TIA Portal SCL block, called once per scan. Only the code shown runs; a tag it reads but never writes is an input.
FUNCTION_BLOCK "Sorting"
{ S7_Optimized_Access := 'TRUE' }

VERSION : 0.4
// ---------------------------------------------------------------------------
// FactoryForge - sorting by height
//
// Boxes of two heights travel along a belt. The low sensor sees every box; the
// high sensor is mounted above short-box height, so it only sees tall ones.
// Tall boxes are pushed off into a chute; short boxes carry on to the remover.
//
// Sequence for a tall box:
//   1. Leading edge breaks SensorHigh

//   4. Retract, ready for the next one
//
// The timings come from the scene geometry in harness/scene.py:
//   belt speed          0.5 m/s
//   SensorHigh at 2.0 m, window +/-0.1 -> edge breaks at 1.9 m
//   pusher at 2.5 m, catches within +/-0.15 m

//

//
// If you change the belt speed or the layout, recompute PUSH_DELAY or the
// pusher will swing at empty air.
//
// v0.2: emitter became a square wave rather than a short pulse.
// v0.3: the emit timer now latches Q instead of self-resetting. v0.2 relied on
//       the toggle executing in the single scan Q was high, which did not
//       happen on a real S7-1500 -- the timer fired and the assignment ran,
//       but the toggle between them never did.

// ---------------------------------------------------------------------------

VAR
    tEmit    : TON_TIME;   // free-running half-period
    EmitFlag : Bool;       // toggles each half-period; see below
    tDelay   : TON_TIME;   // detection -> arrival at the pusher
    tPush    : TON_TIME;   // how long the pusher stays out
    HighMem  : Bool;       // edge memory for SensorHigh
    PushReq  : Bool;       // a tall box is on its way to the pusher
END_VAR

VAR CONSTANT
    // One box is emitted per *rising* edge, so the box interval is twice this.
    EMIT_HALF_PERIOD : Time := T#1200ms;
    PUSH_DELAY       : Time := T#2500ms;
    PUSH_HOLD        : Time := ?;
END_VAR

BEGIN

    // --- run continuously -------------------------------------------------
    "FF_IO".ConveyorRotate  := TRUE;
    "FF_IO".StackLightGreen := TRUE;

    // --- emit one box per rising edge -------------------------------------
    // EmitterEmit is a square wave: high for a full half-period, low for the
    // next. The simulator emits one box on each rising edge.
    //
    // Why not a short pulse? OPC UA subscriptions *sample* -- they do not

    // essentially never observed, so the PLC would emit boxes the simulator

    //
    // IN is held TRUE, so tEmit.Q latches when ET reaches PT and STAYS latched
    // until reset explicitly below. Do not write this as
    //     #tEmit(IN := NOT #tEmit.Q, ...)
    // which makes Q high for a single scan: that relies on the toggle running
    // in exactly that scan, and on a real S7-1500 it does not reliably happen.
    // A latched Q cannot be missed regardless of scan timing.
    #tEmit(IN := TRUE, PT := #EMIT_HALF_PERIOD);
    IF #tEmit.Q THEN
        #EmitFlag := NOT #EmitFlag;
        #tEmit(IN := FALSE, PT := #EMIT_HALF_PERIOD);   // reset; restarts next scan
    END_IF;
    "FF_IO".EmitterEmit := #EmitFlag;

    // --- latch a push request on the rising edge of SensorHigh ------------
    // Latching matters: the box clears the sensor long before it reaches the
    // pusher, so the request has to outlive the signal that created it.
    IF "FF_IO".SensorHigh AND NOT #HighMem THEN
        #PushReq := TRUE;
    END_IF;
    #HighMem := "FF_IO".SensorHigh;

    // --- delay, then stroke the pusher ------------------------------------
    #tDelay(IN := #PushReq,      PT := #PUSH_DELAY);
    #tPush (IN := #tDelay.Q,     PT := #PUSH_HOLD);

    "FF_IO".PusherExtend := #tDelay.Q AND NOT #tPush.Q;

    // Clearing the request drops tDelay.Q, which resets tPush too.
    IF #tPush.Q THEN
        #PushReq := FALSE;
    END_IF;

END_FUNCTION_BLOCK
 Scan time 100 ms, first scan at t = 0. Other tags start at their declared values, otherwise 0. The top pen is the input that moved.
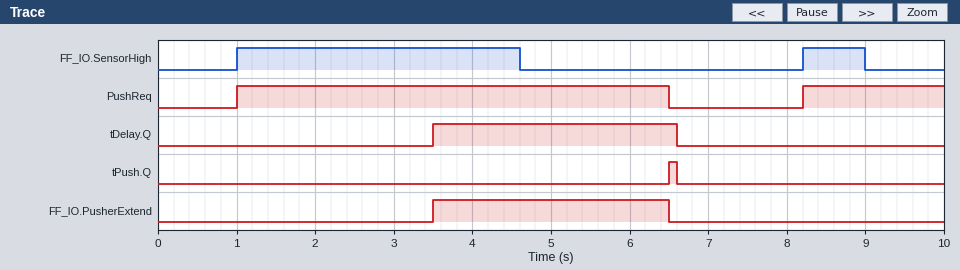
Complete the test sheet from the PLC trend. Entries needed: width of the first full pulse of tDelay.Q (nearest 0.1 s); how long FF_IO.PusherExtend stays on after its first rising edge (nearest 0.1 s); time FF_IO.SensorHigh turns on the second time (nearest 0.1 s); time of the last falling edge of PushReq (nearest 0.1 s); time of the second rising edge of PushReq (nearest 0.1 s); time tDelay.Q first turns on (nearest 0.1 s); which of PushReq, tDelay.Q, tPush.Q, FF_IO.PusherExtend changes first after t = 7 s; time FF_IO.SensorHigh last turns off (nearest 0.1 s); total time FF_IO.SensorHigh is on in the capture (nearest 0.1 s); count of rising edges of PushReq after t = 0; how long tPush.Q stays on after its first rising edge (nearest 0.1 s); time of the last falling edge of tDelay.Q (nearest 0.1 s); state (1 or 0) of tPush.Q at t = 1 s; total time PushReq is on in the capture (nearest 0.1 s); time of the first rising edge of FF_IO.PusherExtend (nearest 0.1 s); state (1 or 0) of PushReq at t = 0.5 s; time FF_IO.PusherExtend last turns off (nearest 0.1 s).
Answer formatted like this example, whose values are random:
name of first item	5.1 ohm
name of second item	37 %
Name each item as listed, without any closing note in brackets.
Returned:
width of the first full pulse of tDelay.Q	3.1 s
how long FF_IO.PusherExtend stays on after its first rising edge	3.0 s
time FF_IO.SensorHigh turns on the second time	8.2 s
time of the last falling edge of PushReq	6.5 s
time of the second rising edge of PushReq	8.2 s
time tDelay.Q first turns on	3.5 s
which of PushReq, tDelay.Q, tPush.Q, FF_IO.PusherExtend changes first after t = 7 s	PushReq
time FF_IO.SensorHigh last turns off	9.0 s
total time FF_IO.SensorHigh is on in the capture	4.4 s
count of rising edges of PushReq after t = 0	2
how long tPush.Q stays on after its first rising edge	0.1 s
time of the last falling edge of tDelay.Q	6.6 s
state (1 or 0) of tPush.Q at t = 1 s	0
total time PushReq is on in the capture	7.3 s
time of the first rising edge of FF_IO.PusherExtend	3.5 s
state (1 or 0) of PushReq at t = 0.5 s	0
time FF_IO.PusherExtend last turns off	6.5 s
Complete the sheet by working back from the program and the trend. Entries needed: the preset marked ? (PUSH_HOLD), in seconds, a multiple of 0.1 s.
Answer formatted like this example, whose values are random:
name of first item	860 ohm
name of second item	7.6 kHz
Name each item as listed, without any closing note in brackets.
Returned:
the preset marked ? (PUSH_HOLD), in seconds, a multiple of 0.1 s	3.0 s
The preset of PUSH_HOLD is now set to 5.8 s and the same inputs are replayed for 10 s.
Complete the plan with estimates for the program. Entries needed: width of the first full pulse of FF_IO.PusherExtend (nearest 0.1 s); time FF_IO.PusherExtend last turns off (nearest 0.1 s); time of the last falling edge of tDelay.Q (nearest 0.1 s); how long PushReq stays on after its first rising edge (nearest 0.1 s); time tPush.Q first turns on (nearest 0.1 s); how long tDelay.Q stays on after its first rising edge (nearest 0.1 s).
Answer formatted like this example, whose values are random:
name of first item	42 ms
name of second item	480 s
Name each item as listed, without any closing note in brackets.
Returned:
width of the first full pulse of FF_IO.PusherExtend	5.8 s
time FF_IO.PusherExtend last turns off	9.3 s
time of the last falling edge of tDelay.Q	9.4 s
how long PushReq stays on after its first rising edge	8.3 s
time tPush.Q first turns on	9.3 s
how long tDelay.Q stays on after its first rising edge	5.9 s
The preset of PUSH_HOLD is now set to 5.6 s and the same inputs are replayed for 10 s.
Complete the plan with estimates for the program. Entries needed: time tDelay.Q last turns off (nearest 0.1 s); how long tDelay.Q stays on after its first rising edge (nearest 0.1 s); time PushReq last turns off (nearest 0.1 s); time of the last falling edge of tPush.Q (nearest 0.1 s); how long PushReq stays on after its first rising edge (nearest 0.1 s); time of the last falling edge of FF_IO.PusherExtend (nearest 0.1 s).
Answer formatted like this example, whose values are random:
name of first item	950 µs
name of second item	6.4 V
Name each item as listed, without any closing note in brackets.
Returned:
time tDelay.Q last turns off	9.2 s
how long tDelay.Q stays on after its first rising edge	5.7 s
time PushReq last turns off	9.1 s
time of the last falling edge of tPush.Q	9.2 s
how long PushReq stays on after its first rising edge	8.1 s
time of the last falling edge of FF_IO.PusherExtend	9.1 s
